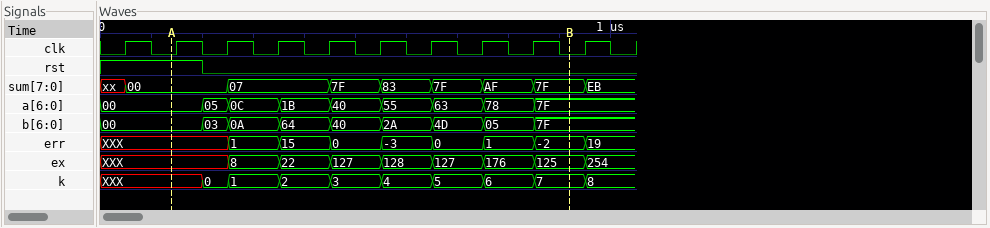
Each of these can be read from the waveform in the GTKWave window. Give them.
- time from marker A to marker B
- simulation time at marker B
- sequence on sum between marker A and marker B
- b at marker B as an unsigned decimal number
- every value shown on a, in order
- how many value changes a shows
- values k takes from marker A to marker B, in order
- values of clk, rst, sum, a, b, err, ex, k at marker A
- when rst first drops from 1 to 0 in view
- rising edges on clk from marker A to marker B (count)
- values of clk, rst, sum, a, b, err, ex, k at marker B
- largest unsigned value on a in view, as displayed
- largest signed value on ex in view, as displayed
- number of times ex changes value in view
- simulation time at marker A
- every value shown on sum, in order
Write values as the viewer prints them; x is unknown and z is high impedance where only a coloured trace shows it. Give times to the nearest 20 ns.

780 ns
920 ns
00, 07, 7F, 83, 7F, AF, 7F
127
00, 05, 0C, 1B, 40, 55, 63, 78, 7F
8
XXX, 0, 1, 2, 3, 4, 5, 6, 7
clk=0, rst=1, sum=00, a=00, b=00, err=XXX, ex=XXX, k=XXX
200 ns
8
clk=0, rst=0, sum=7F, a=7F, b=7F, err=-2, ex=125, k=7
7F
254
8
140 ns
xx, 00, 07, 7F, 83, 7F, AF, 7F, EB
